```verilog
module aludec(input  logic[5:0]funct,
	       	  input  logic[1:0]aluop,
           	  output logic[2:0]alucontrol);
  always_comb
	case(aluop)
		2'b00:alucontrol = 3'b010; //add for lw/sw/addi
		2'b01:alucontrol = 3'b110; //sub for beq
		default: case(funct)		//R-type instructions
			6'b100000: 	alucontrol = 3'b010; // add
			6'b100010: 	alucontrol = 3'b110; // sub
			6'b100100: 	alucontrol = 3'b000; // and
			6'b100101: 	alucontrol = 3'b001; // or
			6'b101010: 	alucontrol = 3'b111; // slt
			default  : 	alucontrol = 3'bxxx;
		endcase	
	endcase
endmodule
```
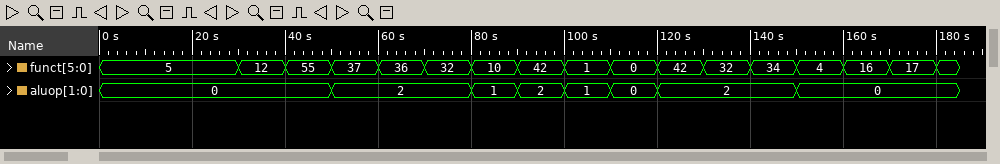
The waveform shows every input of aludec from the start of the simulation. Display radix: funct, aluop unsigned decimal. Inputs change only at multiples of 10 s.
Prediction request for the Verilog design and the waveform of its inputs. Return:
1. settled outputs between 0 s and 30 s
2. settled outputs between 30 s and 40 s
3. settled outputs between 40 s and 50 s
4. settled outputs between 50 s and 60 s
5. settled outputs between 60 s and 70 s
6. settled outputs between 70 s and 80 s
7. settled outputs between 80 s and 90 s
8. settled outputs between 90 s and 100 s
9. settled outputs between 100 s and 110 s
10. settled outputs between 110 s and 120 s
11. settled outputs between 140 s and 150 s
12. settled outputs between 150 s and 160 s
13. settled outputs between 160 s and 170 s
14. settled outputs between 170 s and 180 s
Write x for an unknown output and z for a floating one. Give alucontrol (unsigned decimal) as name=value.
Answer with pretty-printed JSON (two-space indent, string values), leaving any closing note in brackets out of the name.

{
  "settled outputs between 0 s and 30 s": "alucontrol=2",
  "settled outputs between 30 s and 40 s": "alucontrol=2",
  "settled outputs between 40 s and 50 s": "alucontrol=2",
  "settled outputs between 50 s and 60 s": "alucontrol=1",
  "settled outputs between 60 s and 70 s": "alucontrol=0",
  "settled outputs between 70 s and 80 s": "alucontrol=2",
  "settled outputs between 80 s and 90 s": "alucontrol=6",
  "settled outputs between 90 s and 100 s": "alucontrol=7",
  "settled outputs between 100 s and 110 s": "alucontrol=6",
  "settled outputs between 110 s and 120 s": "alucontrol=2",
  "settled outputs between 140 s and 150 s": "alucontrol=6",
  "settled outputs between 150 s and 160 s": "alucontrol=2",
  "settled outputs between 160 s and 170 s": "alucontrol=2",
  "settled outputs between 170 s and 180 s": "alucontrol=2"
}
